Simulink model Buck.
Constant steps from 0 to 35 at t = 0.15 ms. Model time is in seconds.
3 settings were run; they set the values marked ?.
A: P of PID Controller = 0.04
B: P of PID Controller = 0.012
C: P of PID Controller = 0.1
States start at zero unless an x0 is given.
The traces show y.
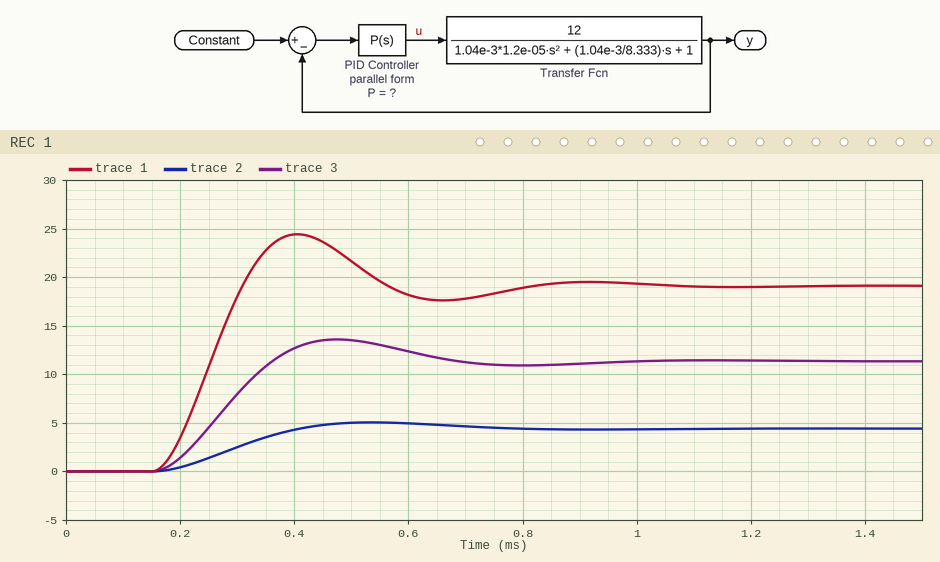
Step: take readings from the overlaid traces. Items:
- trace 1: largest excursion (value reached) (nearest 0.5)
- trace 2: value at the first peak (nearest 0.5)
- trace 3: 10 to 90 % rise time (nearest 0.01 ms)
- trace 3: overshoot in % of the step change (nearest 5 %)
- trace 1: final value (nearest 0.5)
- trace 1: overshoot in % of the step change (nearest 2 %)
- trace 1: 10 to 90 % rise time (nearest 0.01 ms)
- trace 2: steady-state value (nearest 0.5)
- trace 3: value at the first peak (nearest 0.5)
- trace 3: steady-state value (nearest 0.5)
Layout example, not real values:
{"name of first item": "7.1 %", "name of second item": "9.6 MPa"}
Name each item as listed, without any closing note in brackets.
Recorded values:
{"trace 1: largest excursion (value reached)": "24.5", "trace 2: value at the first peak": "5.0", "trace 3: 10 to 90 % rise time": "0.14 ms", "trace 3: overshoot in % of the step change": "20 %", "trace 1: final value": "19.0", "trace 1: overshoot in % of the step change": "28 %", "trace 1: 10 to 90 % rise time": "0.11 ms", "trace 2: steady-state value": "4.5", "trace 3: value at the first peak": "13.5", "trace 3: steady-state value": "11.5"}
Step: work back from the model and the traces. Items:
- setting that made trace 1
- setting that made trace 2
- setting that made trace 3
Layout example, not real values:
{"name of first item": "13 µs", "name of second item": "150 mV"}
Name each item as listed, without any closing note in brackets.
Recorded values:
{"setting that made trace 1": "C", "setting that made trace 2": "B", "setting that made trace 3": "A"}
